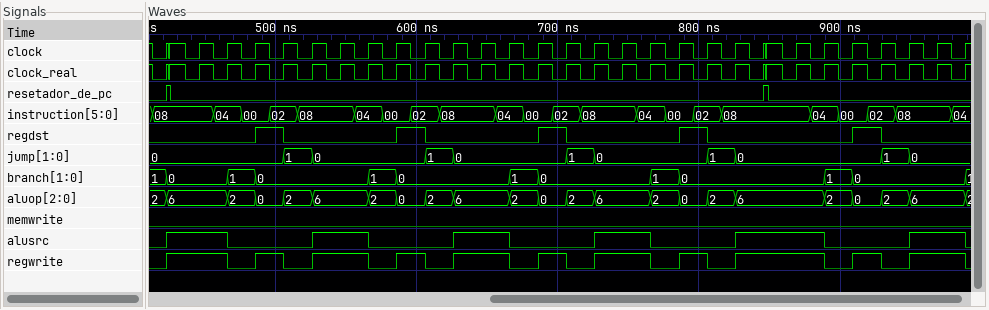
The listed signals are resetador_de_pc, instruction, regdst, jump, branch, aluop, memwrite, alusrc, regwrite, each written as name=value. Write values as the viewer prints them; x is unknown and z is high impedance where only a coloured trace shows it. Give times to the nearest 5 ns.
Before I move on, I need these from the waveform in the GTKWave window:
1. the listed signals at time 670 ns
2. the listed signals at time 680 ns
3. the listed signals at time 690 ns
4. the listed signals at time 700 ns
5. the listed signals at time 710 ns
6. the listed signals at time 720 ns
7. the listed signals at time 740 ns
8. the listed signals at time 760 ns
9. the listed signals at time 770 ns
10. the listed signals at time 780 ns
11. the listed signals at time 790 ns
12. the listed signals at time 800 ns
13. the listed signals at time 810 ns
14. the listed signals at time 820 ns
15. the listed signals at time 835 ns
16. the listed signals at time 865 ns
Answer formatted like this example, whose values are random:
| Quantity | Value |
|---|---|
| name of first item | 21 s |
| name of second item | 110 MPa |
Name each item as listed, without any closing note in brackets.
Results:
| Quantity | Value |
|---|---|
| the listed signals at time 670 ns | resetador_de_pc=0, instruction=04, regdst=0, jump=0, branch=1, aluop=2, memwrite=0, alusrc=0, regwrite=0 |
| the listed signals at time 680 ns | resetador_de_pc=0, instruction=00, regdst=0, jump=0, branch=1, aluop=2, memwrite=0, alusrc=0, regwrite=0 |
| the listed signals at time 690 ns | resetador_de_pc=0, instruction=00, regdst=1, jump=0, branch=0, aluop=0, memwrite=0, alusrc=0, regwrite=1 |
| the listed signals at time 700 ns | resetador_de_pc=0, instruction=02, regdst=1, jump=0, branch=0, aluop=0, memwrite=0, alusrc=0, regwrite=1 |
| the listed signals at time 710 ns | resetador_de_pc=0, instruction=02, regdst=0, jump=1, branch=0, aluop=2, memwrite=0, alusrc=0, regwrite=0 |
| the listed signals at time 720 ns | resetador_de_pc=0, instruction=08, regdst=0, jump=1, branch=0, aluop=2, memwrite=0, alusrc=0, regwrite=0 |
| the listed signals at time 740 ns | resetador_de_pc=0, instruction=08, regdst=0, jump=0, branch=0, aluop=6, memwrite=0, alusrc=1, regwrite=1 |
| the listed signals at time 760 ns | resetador_de_pc=0, instruction=04, regdst=0, jump=0, branch=0, aluop=6, memwrite=0, alusrc=1, regwrite=1 |
| the listed signals at time 770 ns | resetador_de_pc=0, instruction=04, regdst=0, jump=0, branch=1, aluop=2, memwrite=0, alusrc=0, regwrite=0 |
| the listed signals at time 780 ns | resetador_de_pc=0, instruction=00, regdst=0, jump=0, branch=1, aluop=2, memwrite=0, alusrc=0, regwrite=0 |
| the listed signals at time 790 ns | resetador_de_pc=0, instruction=00, regdst=1, jump=0, branch=0, aluop=0, memwrite=0, alusrc=0, regwrite=1 |
| the listed signals at time 800 ns | resetador_de_pc=0, instruction=02, regdst=1, jump=0, branch=0, aluop=0, memwrite=0, alusrc=0, regwrite=1 |
| the listed signals at time 810 ns | resetador_de_pc=0, instruction=02, regdst=0, jump=1, branch=0, aluop=2, memwrite=0, alusrc=0, regwrite=0 |
| the listed signals at time 820 ns | resetador_de_pc=0, instruction=08, regdst=0, jump=1, branch=0, aluop=2, memwrite=0, alusrc=0, regwrite=0 |
| the listed signals at time 835 ns | resetador_de_pc=0, instruction=08, regdst=0, jump=0, branch=0, aluop=6, memwrite=0, alusrc=1, regwrite=1 |
| the listed signals at time 865 ns | resetador_de_pc=0, instruction=08, regdst=0, jump=0, branch=0, aluop=6, memwrite=0, alusrc=1, regwrite=1 |
